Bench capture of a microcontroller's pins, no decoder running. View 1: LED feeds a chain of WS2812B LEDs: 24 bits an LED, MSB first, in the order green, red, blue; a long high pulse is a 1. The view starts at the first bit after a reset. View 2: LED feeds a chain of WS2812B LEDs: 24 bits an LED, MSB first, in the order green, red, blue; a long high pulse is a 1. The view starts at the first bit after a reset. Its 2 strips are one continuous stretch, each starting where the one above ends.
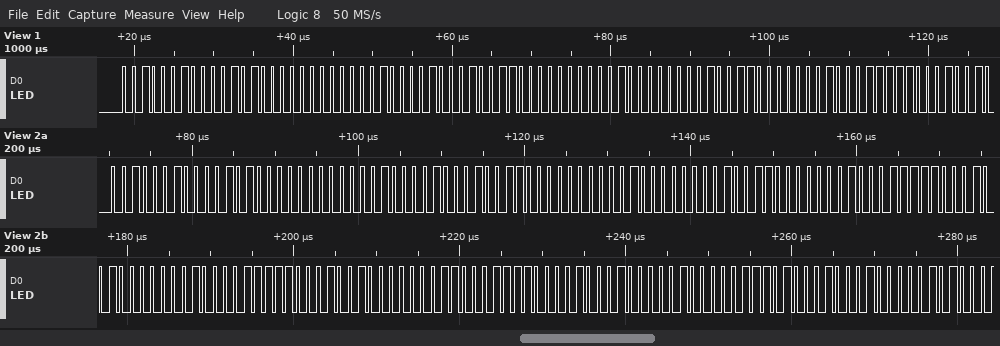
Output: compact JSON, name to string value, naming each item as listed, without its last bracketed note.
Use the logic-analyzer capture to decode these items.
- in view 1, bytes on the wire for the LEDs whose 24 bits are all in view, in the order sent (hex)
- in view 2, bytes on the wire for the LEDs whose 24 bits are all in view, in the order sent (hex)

{"in view 1, bytes on the wire for the LEDs whose 24 bits are all in view, in the order sent": "22 14 00 21 13 00 20 13 01", "in view 2, bytes on the wire for the LEDs whose 24 bits are all in view, in the order sent": "22 14 00 21 13 00 20 13 01 1F 12 02 1F 12 03 1E 11 04 1D 11 05"}
